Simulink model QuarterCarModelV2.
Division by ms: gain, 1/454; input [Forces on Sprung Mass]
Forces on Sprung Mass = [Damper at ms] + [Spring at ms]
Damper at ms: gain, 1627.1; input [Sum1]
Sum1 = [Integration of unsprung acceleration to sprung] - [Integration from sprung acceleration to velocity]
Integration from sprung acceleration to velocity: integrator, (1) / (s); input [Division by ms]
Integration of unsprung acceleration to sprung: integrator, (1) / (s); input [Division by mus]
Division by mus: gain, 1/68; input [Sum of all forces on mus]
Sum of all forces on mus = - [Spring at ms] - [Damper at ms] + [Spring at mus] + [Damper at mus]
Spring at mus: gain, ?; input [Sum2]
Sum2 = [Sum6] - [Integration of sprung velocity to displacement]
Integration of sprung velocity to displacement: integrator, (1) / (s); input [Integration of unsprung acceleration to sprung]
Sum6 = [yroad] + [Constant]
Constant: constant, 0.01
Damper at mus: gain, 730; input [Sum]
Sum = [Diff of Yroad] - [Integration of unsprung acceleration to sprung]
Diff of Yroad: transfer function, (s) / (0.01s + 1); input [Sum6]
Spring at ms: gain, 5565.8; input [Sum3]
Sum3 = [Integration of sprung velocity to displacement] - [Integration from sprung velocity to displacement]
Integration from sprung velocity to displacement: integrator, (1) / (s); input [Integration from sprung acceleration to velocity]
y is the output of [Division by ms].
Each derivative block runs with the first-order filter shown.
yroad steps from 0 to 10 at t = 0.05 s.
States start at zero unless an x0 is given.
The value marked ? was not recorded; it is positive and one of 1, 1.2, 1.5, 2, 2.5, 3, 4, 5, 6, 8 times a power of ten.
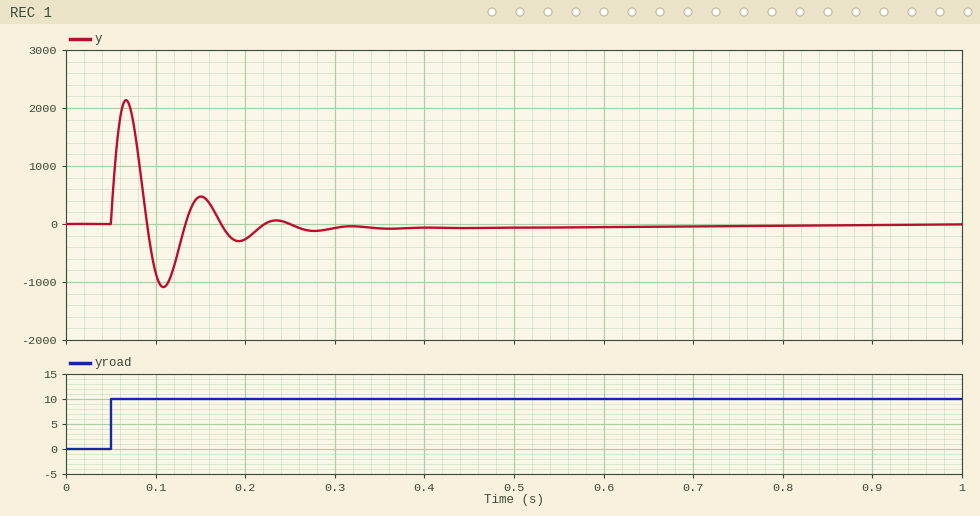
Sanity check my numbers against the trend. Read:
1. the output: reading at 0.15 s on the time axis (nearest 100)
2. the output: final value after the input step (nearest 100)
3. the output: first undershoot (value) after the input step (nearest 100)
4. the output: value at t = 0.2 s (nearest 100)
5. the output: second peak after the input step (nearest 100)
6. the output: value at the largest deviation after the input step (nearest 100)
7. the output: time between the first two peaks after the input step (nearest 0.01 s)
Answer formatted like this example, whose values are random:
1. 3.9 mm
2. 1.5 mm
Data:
1. 500
2. 0
3. -1100
4. -300
5. 500
6. 2100
7. 0.08 s
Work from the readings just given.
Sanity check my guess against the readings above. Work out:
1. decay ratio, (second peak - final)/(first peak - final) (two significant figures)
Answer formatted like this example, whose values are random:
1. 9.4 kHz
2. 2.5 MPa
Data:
1. 0.24
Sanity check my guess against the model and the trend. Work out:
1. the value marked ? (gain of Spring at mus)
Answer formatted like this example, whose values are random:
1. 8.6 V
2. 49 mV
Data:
1. 400000
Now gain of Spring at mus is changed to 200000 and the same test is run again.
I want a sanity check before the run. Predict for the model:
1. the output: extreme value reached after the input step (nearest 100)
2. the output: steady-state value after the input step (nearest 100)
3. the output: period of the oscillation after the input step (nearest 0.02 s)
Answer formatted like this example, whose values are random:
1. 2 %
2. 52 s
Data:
1. 1400
2. 0
3. 0.12 s
